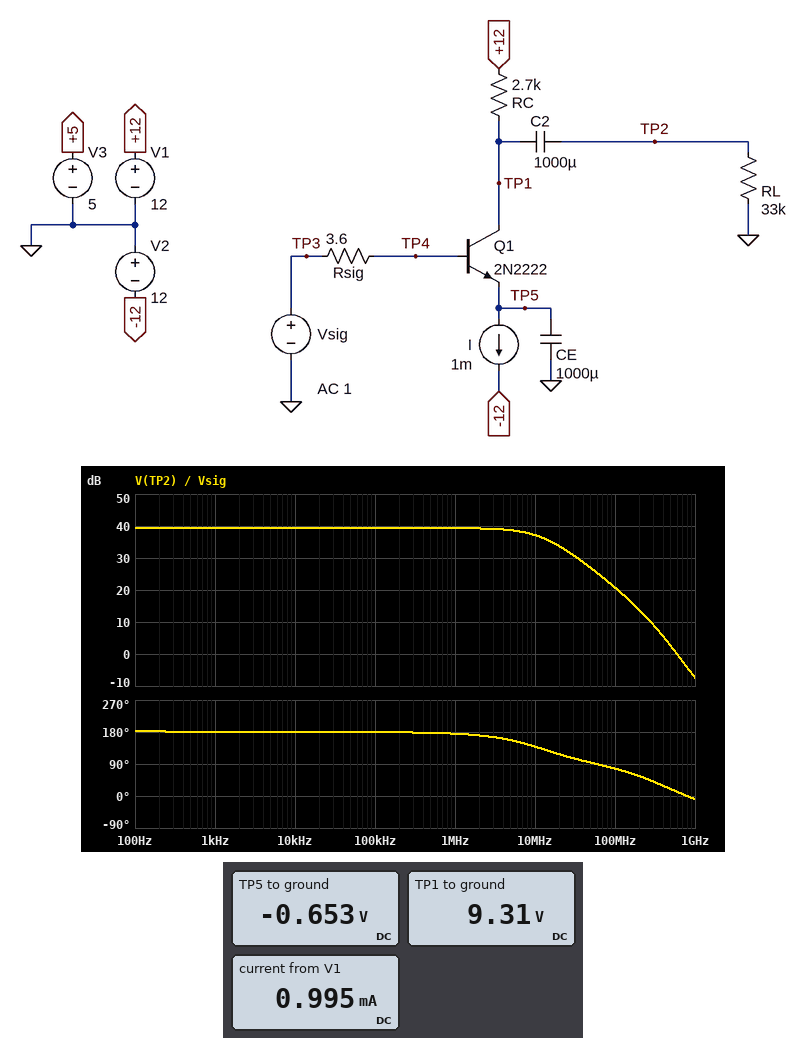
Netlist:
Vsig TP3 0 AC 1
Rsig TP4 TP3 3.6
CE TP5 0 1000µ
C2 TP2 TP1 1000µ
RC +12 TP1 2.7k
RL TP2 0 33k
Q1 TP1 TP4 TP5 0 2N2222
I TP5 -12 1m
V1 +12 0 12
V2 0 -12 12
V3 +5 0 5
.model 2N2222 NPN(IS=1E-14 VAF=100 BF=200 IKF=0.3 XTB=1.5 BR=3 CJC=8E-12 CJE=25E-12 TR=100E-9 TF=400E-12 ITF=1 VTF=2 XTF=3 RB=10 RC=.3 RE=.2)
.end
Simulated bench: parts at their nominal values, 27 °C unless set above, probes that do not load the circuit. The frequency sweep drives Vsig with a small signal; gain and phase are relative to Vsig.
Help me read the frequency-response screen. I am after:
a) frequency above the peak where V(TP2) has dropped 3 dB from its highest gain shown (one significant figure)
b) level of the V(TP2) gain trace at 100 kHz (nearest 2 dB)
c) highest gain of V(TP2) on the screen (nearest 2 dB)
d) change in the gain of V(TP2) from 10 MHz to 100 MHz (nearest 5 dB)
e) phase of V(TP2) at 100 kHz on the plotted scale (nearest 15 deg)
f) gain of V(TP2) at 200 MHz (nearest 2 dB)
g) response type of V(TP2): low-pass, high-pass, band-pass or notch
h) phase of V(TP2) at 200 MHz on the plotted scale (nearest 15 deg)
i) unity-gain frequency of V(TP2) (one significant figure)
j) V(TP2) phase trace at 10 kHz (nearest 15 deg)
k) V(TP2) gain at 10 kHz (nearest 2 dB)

10 MHz
40 dB
40 dB
-15 dB
180 deg
14 dB
low-pass
60 deg
600 MHz
180 deg
40 dB
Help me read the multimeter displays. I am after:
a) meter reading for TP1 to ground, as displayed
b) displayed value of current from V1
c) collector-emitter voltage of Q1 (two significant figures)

9.31 V
0.995 mA
10 V
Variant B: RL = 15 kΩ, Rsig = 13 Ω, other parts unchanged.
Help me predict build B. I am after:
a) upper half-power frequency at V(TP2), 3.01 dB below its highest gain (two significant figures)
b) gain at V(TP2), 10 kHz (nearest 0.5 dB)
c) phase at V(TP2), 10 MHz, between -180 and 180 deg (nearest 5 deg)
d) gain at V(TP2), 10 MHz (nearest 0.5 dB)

11 MHz
38.5 dB
135 deg
36.0 dB
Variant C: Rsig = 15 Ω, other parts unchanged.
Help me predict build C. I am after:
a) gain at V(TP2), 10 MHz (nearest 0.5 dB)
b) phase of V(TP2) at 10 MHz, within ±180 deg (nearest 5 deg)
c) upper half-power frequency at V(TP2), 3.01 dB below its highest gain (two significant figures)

36.0 dB
130 deg
9.4 MHz
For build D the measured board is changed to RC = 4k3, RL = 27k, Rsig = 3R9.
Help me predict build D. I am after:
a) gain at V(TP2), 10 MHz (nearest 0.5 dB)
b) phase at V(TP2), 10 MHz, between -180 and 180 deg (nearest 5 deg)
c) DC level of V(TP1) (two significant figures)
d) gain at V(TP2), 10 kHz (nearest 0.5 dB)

38.5 dB
125 deg
7.7 V
42.5 dB
